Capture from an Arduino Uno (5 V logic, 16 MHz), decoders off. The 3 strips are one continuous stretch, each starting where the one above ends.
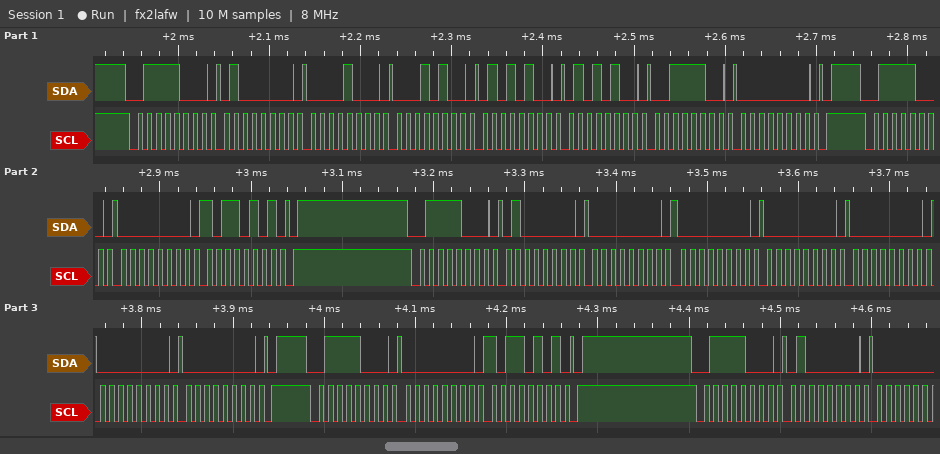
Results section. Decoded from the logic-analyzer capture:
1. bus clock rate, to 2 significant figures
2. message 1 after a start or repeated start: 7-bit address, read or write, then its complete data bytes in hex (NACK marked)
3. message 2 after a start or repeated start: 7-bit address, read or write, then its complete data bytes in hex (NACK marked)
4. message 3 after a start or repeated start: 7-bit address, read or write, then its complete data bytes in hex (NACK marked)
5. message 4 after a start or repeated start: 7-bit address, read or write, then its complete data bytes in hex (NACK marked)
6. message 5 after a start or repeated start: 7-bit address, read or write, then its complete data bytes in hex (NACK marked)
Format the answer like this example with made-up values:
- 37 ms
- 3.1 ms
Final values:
- 100 kHz
- 0x3C write: 40 08 14 54 54 3C 00
- 0x3C write: 00 B5
- 0x3C write: 40 00 00 00 00 00 00
- 0x3C write: 00 B5
- 0x3C write: 40
